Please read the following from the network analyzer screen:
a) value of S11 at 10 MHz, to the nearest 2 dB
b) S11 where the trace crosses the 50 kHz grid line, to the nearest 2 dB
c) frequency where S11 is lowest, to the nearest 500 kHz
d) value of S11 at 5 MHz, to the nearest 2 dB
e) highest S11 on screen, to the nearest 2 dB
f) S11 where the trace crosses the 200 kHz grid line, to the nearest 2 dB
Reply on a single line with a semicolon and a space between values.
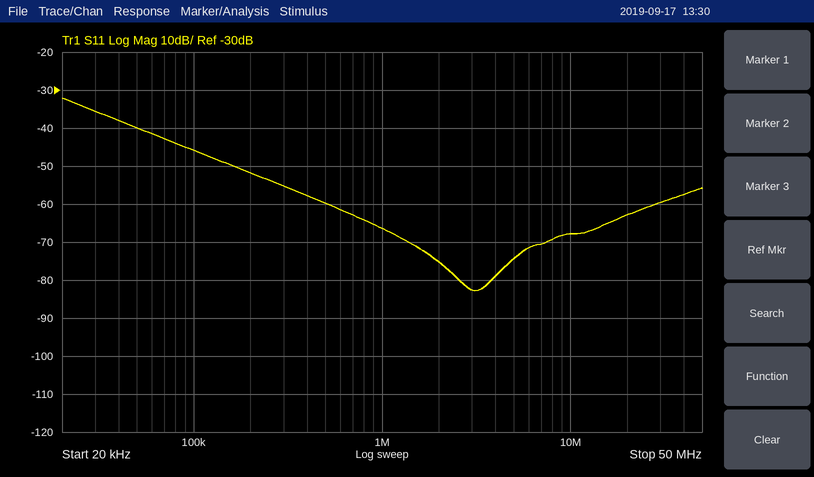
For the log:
-68 dB; -40 dB; 3.0 MHz; -74 dB; -32 dB; -52 dB
